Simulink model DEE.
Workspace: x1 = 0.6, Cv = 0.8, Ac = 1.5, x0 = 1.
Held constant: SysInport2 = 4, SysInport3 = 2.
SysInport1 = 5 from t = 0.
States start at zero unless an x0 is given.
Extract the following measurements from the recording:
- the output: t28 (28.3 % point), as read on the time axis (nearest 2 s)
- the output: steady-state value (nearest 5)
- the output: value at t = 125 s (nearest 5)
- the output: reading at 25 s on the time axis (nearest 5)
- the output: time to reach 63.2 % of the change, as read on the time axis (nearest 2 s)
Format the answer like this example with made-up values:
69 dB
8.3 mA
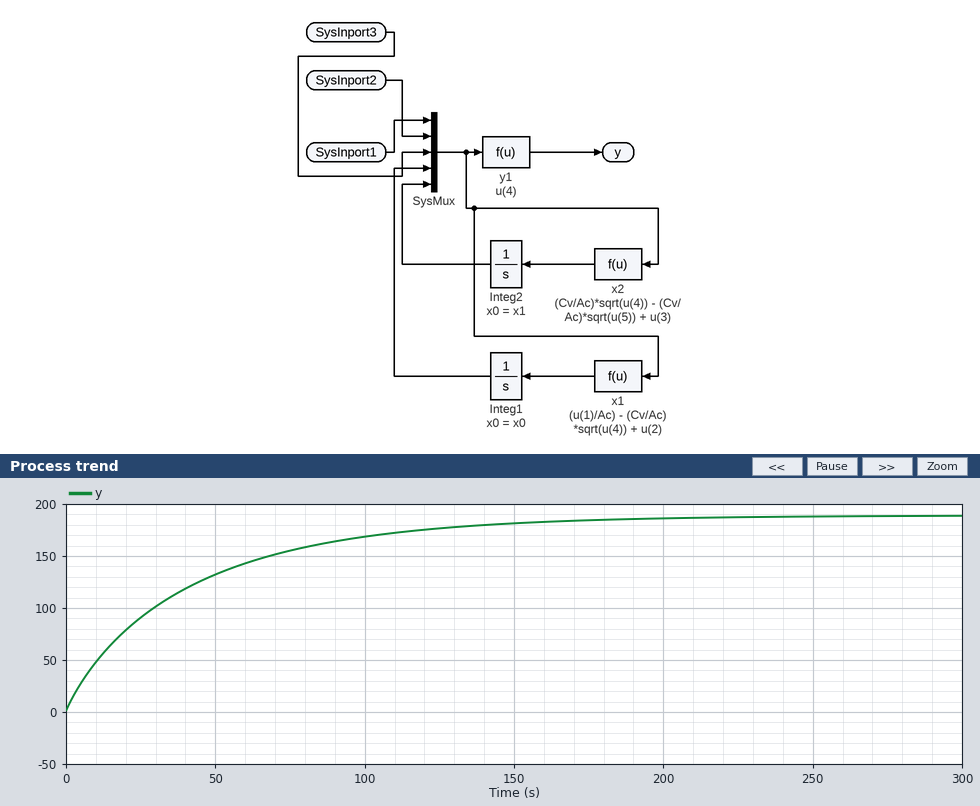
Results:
12 s
190
175
90
40 s
